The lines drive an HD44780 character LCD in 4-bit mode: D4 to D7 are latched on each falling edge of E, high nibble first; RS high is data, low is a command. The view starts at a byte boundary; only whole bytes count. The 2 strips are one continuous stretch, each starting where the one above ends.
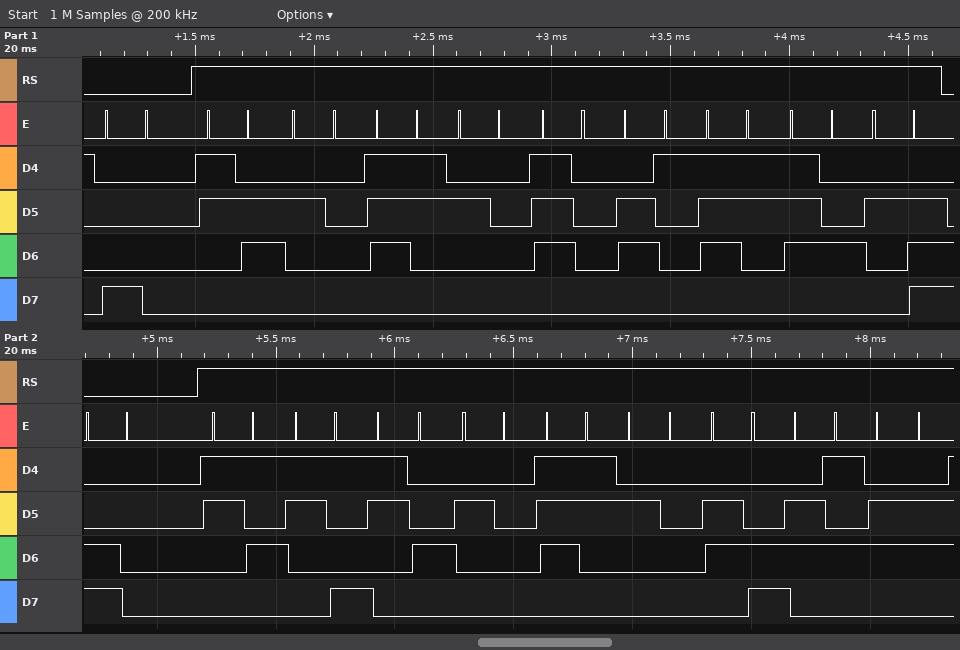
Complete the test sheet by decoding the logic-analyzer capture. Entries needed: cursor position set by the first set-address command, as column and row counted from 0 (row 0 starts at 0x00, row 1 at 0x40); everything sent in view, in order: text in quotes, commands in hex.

column 0, row 0
0x80 "6 s past." 0xC0 "594 s lef"
